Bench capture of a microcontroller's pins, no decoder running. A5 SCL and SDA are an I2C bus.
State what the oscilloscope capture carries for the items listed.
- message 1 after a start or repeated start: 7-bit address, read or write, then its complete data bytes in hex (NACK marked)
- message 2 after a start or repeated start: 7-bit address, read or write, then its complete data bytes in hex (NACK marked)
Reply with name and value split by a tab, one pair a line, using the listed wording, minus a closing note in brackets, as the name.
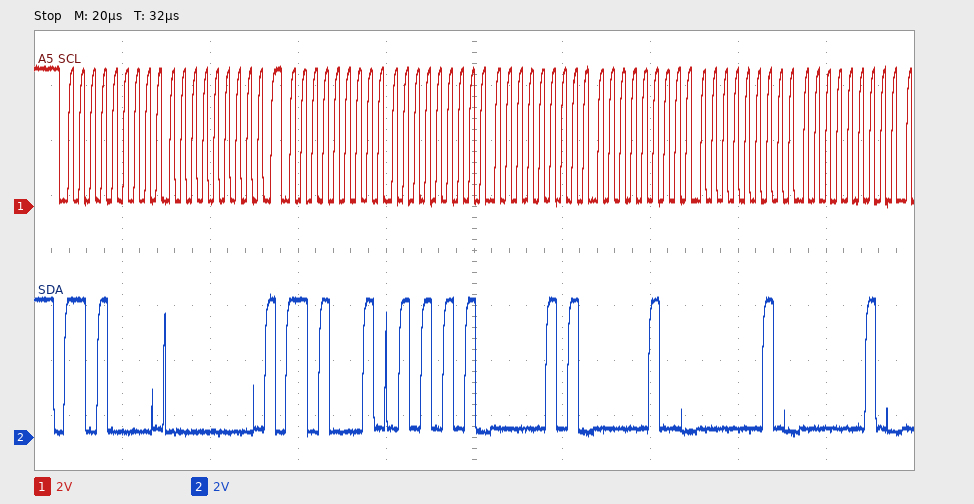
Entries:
message 1 after a start or repeated start: 7-bit address, read or write, then its complete data bytes in hex	0x68 write: 00
message 2 after a start or repeated start: 7-bit address, read or write, then its complete data bytes in hex	0x68 read: 55 05 04 02 02
